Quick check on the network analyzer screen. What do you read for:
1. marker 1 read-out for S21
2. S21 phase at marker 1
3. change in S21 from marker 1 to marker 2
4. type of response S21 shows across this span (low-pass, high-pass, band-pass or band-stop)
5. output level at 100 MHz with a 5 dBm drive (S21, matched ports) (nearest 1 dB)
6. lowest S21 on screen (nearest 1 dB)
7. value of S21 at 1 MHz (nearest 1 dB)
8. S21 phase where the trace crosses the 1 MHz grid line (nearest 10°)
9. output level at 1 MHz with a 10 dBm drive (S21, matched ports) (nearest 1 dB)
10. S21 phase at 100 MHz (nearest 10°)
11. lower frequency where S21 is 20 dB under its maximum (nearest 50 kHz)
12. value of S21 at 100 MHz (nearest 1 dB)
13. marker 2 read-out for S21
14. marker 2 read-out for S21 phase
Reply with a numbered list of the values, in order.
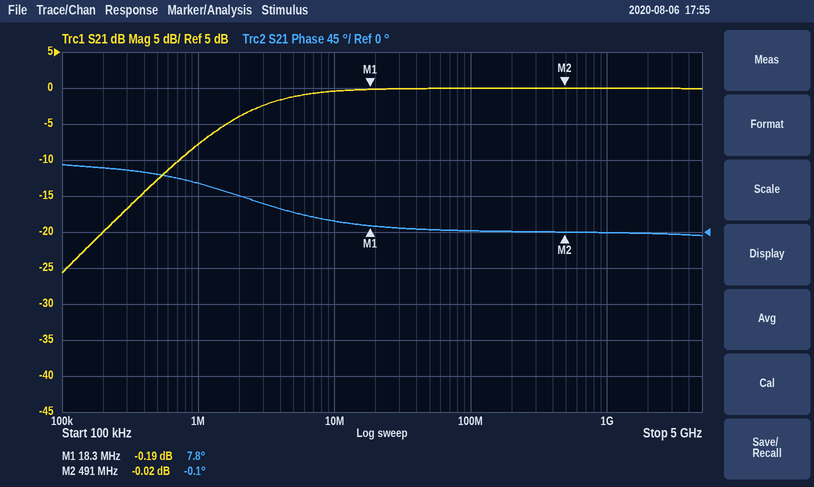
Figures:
1. -0.19 dB
2. 7.8°
3. 0.17 dB
4. high-pass
5. 5 dBm
6. -26 dB
7. -8 dB
8. 60°
9. 2 dBm
10. 0°
11. 200 kHz
12. 0 dB
13. -0.02 dB
14. -0.1°
